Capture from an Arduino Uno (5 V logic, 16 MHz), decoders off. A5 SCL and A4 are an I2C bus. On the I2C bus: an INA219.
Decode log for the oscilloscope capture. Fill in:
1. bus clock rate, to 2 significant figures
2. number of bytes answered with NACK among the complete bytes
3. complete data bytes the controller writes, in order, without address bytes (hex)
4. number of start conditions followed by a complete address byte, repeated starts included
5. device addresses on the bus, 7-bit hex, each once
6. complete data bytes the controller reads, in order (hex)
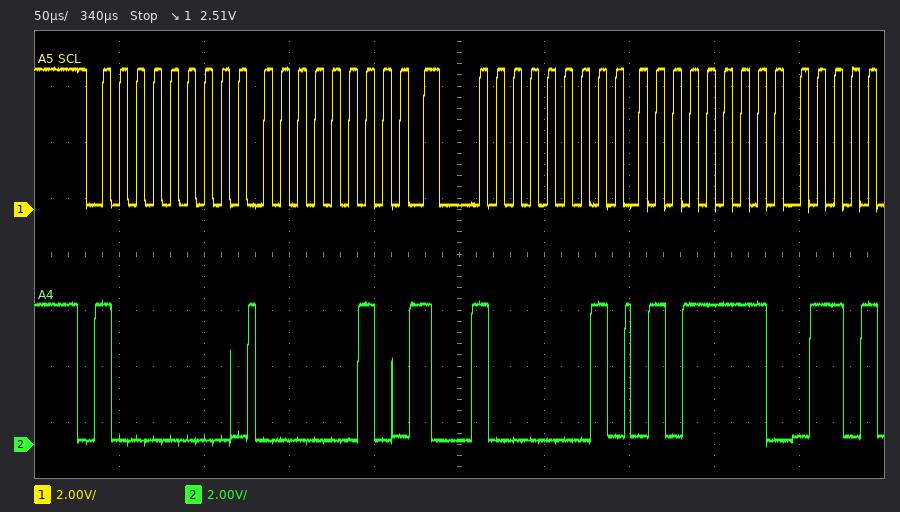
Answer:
100 kHz
0
02
2
0x40
5F
